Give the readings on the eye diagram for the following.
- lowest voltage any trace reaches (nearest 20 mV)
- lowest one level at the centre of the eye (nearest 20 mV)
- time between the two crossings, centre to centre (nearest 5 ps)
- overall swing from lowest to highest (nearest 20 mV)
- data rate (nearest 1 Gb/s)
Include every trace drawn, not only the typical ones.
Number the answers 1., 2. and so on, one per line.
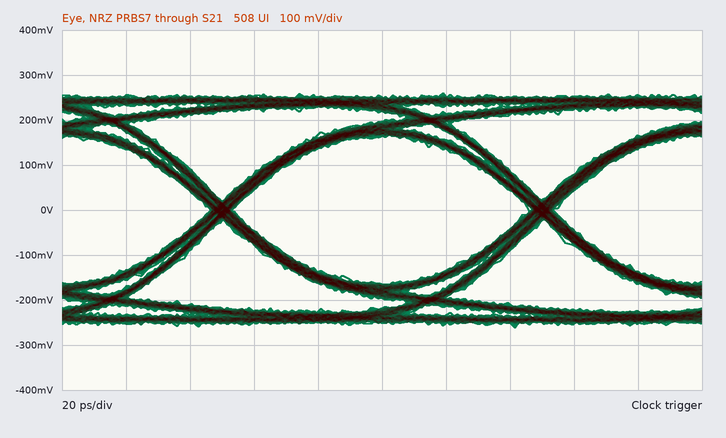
1. -260 mV
2. 160 mV
3. 100 ps
4. 520 mV
5. 10 Gb/s
